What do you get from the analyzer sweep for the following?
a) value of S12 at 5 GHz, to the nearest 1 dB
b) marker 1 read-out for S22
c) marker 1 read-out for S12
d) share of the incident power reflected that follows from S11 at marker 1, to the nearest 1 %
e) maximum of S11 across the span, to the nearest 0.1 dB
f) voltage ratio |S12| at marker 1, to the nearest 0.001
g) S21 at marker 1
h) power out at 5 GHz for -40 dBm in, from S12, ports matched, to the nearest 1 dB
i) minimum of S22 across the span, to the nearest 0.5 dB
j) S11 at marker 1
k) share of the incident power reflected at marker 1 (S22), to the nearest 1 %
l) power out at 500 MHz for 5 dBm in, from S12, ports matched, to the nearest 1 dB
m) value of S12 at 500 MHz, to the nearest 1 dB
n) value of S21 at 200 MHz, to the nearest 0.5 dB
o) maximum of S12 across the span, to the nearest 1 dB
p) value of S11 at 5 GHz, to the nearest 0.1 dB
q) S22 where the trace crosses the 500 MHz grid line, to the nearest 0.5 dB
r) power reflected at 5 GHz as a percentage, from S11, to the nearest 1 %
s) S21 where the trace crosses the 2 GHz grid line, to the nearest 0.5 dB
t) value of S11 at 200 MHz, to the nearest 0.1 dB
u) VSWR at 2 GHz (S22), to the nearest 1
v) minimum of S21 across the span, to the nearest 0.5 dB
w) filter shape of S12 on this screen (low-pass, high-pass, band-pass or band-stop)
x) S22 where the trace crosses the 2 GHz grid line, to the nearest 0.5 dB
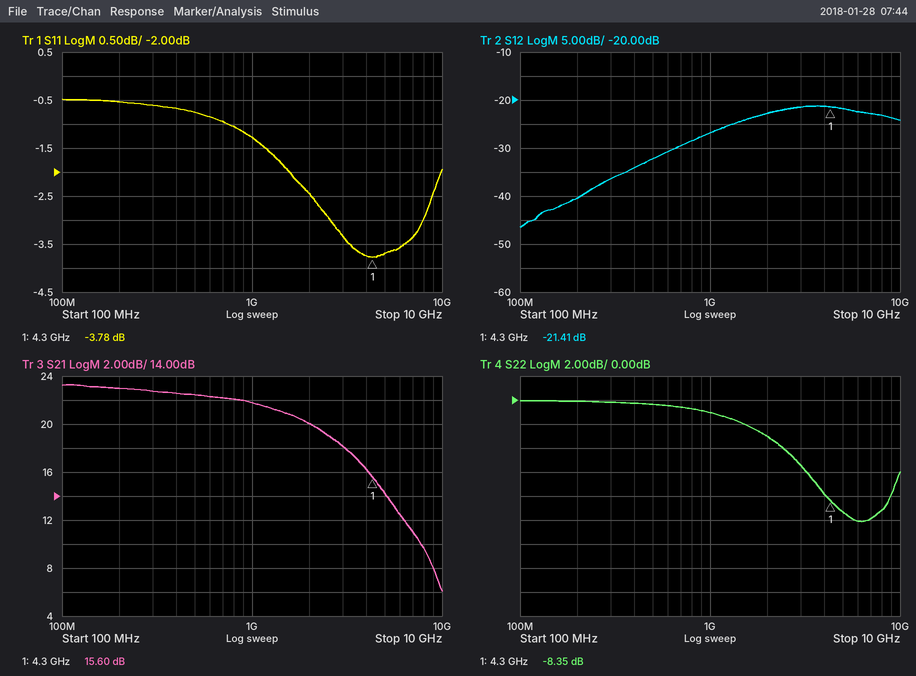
-22 dB
-8.35 dB
-21.41 dB
42 %
-0.5 dB
0.085
15.60 dB
-62 dBm
-10.0 dB
-3.78 dB
15 %
-27 dBm
-32 dB
23.0 dB
-21 dB
-3.7 dB
-0.5 dB
43 %
20.0 dB
-0.5 dB
6
6.0 dB
high-pass
-3.0 dB
